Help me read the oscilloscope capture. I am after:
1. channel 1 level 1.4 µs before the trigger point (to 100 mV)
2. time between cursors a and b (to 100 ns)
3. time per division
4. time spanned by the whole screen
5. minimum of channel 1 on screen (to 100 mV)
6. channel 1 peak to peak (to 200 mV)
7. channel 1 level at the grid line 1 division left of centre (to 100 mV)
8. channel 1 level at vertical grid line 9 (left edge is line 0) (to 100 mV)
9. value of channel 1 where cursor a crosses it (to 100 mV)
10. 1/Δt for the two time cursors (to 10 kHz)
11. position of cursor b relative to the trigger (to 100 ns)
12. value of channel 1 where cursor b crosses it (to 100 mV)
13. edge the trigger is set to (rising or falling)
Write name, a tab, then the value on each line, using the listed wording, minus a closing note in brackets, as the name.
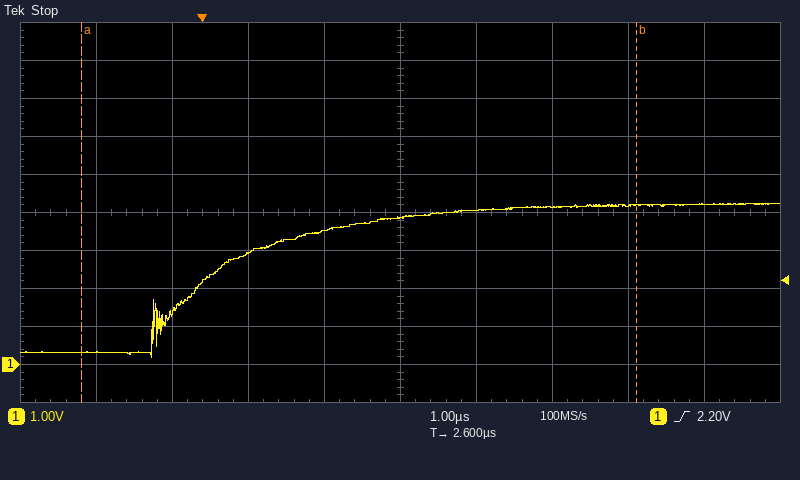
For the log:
channel 1 level 1.4 µs before the trigger point	300 mV
time between cursors a and b	7.3 µs
time per division	1 µs
time spanned by the whole screen	10 µs
minimum of channel 1 on screen	200 mV
channel 1 peak to peak	4.0 V
channel 1 level at the grid line 1 division left of centre	3.5 V
channel 1 level at vertical grid line 9 (left edge is line 0)	4.2 V
value of channel 1 where cursor a crosses it	300 mV
1/Δt for the two time cursors	140 kHz
position of cursor b relative to the trigger	+5.7 µs
value of channel 1 where cursor b crosses it	4.2 V
edge the trigger is set to	rising
